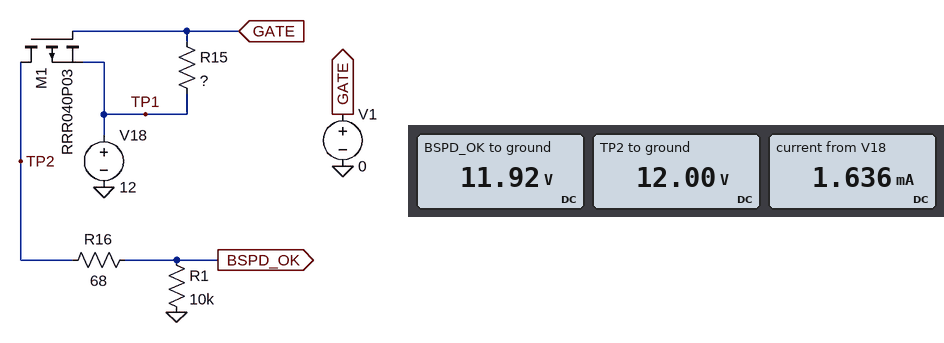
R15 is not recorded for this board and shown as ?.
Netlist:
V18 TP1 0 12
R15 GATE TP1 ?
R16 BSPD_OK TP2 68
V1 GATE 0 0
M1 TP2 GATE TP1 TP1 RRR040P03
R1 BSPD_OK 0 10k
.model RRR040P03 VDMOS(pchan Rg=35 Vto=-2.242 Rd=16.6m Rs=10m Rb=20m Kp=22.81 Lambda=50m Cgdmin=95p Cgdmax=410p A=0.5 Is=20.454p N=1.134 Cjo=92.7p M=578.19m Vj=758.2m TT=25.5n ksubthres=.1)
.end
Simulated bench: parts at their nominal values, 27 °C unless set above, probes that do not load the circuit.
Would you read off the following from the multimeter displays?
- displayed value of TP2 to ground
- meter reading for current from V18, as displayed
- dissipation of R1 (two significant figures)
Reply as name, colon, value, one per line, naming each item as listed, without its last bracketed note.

displayed value of TP2 to ground: 12.00 V
meter reading for current from V18, as displayed: 1.636 mA
dissipation of R1: 14 mW
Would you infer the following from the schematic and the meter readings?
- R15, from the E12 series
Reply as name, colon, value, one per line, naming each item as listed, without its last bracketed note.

R15, from the E12 series: 27 kΩ
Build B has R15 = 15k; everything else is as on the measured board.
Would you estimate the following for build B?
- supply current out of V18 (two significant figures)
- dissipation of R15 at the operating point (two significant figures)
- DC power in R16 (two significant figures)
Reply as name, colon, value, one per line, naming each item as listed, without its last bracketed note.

supply current out of V18: 2.0 mA
dissipation of R15 at the operating point: 9.6 mW
DC power in R16: 97 µW
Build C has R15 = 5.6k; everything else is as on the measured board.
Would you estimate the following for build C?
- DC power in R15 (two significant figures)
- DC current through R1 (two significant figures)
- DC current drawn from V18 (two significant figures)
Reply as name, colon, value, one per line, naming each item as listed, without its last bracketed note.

DC power in R15: 26 mW
DC current through R1: 1.2 mA
DC current drawn from V18: 3.3 mA
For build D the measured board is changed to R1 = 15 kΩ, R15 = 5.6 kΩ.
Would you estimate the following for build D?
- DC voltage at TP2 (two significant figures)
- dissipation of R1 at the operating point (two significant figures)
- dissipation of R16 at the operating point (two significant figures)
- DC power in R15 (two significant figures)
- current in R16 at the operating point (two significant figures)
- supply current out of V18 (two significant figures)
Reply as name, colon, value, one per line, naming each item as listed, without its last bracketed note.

DC voltage at TP2: 12 V
dissipation of R1 at the operating point: 9.5 mW
dissipation of R16 at the operating point: 43 µW
DC power in R15: 26 mW
current in R16 at the operating point: 800 µA
supply current out of V18: 2.9 mA
